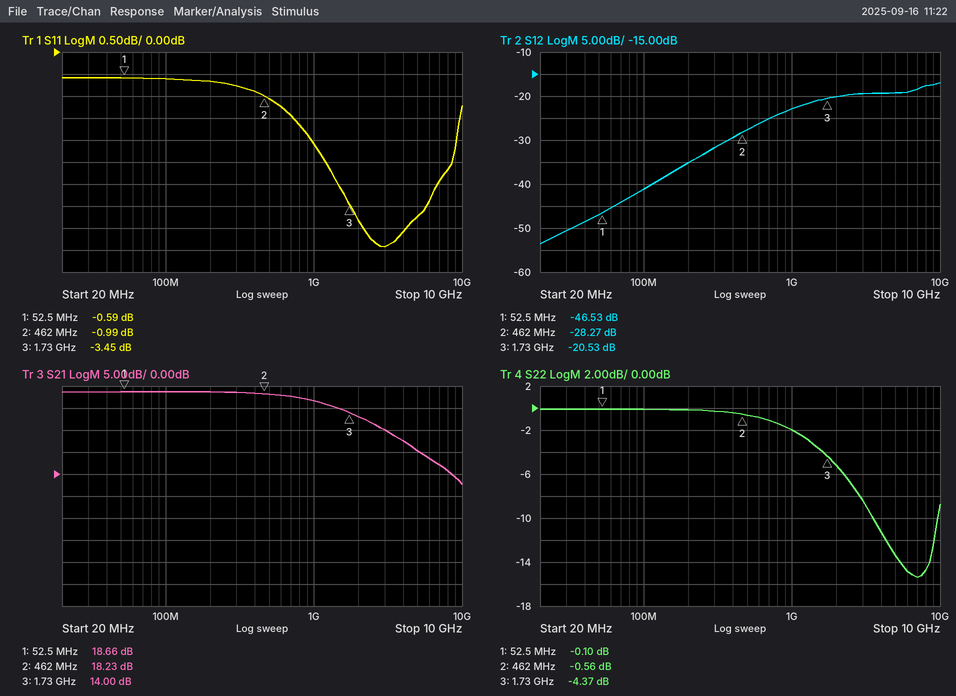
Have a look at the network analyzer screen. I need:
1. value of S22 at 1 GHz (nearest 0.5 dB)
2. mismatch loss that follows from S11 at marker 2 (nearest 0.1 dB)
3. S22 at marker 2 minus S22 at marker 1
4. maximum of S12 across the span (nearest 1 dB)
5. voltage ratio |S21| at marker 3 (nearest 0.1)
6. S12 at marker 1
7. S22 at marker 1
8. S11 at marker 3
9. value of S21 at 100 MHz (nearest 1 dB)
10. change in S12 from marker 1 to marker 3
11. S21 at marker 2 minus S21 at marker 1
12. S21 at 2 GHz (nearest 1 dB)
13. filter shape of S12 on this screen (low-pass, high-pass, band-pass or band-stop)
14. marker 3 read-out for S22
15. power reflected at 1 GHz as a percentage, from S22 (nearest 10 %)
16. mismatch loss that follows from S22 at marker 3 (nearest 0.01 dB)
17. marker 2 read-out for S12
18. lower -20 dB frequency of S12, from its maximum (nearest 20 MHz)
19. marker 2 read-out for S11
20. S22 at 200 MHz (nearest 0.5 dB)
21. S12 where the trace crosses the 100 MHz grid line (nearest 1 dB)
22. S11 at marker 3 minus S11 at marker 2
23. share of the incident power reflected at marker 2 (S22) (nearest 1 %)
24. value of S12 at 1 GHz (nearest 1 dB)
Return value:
-2.0 dB
6.9 dB
-0.46 dB
-17 dB
5.0
-46.53 dB
-0.10 dB
-3.45 dB
19 dB
26.00 dB
-0.43 dB
13 dB
high-pass
-4.37 dB
60 %
1.98 dB
-28.27 dB
160 MHz
-0.99 dB
0.0 dB
-41 dB
-2.46 dB
88 %
-23 dB
